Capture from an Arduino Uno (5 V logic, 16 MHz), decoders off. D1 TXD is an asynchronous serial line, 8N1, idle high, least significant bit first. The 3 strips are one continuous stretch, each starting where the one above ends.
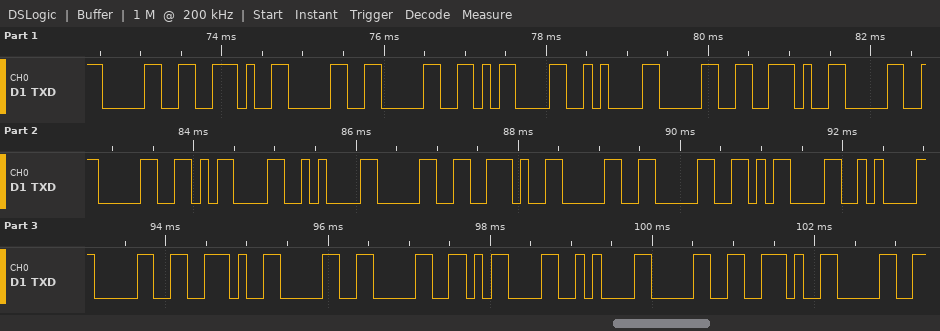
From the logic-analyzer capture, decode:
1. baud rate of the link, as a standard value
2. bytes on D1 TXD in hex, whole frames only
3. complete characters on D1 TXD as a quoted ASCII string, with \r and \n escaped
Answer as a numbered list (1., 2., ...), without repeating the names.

1. 9600 baud
2. 30 2E 30 30 0D 0A 30 2E 30 30 0D 0A 30 2E 30 30 0D 0A 30 2E 30 30 0D 0A 30 2E 30
3. "0.00\r\n0.00\r\n0.00\r\n0.00\r\n0.0"
